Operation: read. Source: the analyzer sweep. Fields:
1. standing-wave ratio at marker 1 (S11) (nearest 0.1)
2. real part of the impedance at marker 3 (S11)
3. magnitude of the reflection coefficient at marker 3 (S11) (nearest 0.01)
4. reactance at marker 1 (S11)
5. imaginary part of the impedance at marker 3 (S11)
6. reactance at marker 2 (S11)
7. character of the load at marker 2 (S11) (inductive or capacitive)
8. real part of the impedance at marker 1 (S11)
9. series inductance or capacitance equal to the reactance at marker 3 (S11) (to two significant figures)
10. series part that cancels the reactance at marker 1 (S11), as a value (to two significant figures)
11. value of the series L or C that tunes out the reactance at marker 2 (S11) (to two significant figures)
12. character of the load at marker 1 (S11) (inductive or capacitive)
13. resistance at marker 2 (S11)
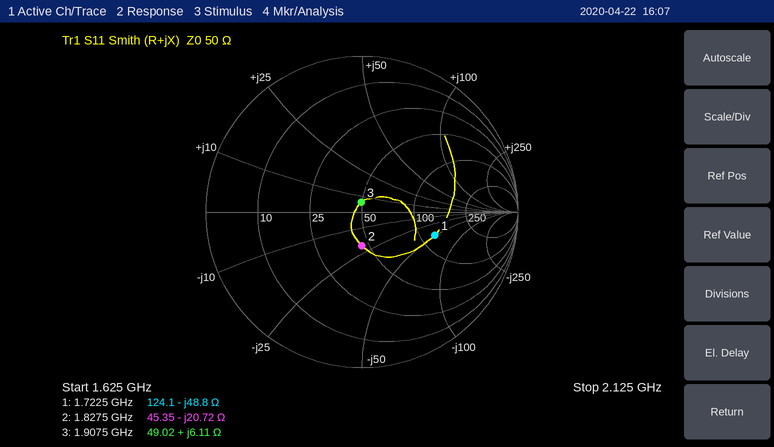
2.9
49.02 Ω
0.06
-48.8 Ω
+6.11 Ω
-20.72 Ω
capacitive
124.1 Ω
510 pH
4.5 nH
1.8 nH
capacitive
45.35 Ω
